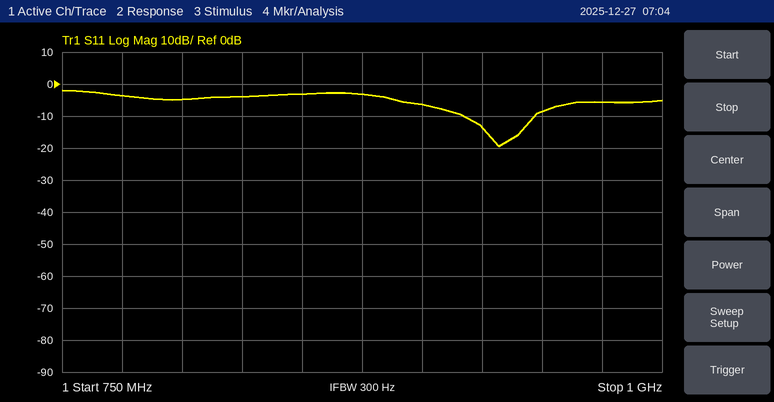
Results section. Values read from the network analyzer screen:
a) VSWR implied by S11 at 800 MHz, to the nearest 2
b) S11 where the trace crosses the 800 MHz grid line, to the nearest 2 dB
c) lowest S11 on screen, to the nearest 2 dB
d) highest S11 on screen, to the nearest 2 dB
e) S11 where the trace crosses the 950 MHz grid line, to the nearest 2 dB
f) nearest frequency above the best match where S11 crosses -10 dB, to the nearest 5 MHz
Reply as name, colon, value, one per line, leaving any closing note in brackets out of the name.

VSWR implied by S11 at 800 MHz, to the nearest 2: 4
S11 where the trace crosses the 800 MHz grid line, to the nearest 2 dB: -4 dB
lowest S11 on screen, to the nearest 2 dB: -20 dB
highest S11 on screen, to the nearest 2 dB: -2 dB
S11 where the trace crosses the 950 MHz grid line, to the nearest 2 dB: -8 dB
nearest frequency above the best match where S11 crosses -10 dB, to the nearest 5 MHz: 945 MHz
